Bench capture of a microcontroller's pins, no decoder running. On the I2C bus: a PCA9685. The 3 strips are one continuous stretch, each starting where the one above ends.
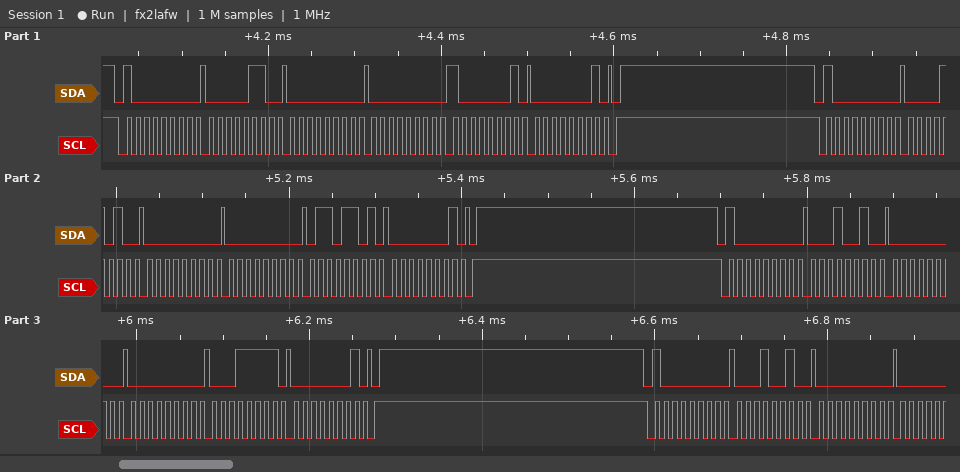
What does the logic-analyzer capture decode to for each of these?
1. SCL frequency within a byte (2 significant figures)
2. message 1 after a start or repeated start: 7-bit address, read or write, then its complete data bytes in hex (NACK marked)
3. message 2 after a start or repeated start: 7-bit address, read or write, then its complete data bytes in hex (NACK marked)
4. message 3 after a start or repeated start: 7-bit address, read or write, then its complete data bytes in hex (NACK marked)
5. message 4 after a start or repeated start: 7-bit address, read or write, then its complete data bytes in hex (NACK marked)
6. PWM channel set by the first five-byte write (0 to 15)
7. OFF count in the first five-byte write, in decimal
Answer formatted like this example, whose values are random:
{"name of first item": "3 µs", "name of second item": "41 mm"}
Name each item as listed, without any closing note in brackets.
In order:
{"SCL frequency within a byte": "100 kHz", "message 1 after a start or repeated start: 7-bit address, read or write, then its complete data bytes in hex": "0x40 write: 06 00 00 81 01", "message 2 after a start or repeated start: 7-bit address, read or write, then its complete data bytes in hex": "0x40 write: 0A 00 00 6D 01", "message 3 after a start or repeated start: 7-bit address, read or write, then its complete data bytes in hex": "0x40 write: 12 00 00 1F 01", "message 4 after a start or repeated start: 7-bit address, read or write, then its complete data bytes in hex": "0x40 write: 12 00", "PWM channel set by the first five-byte write": "0", "OFF count in the first five-byte write, in decimal": "385"}
